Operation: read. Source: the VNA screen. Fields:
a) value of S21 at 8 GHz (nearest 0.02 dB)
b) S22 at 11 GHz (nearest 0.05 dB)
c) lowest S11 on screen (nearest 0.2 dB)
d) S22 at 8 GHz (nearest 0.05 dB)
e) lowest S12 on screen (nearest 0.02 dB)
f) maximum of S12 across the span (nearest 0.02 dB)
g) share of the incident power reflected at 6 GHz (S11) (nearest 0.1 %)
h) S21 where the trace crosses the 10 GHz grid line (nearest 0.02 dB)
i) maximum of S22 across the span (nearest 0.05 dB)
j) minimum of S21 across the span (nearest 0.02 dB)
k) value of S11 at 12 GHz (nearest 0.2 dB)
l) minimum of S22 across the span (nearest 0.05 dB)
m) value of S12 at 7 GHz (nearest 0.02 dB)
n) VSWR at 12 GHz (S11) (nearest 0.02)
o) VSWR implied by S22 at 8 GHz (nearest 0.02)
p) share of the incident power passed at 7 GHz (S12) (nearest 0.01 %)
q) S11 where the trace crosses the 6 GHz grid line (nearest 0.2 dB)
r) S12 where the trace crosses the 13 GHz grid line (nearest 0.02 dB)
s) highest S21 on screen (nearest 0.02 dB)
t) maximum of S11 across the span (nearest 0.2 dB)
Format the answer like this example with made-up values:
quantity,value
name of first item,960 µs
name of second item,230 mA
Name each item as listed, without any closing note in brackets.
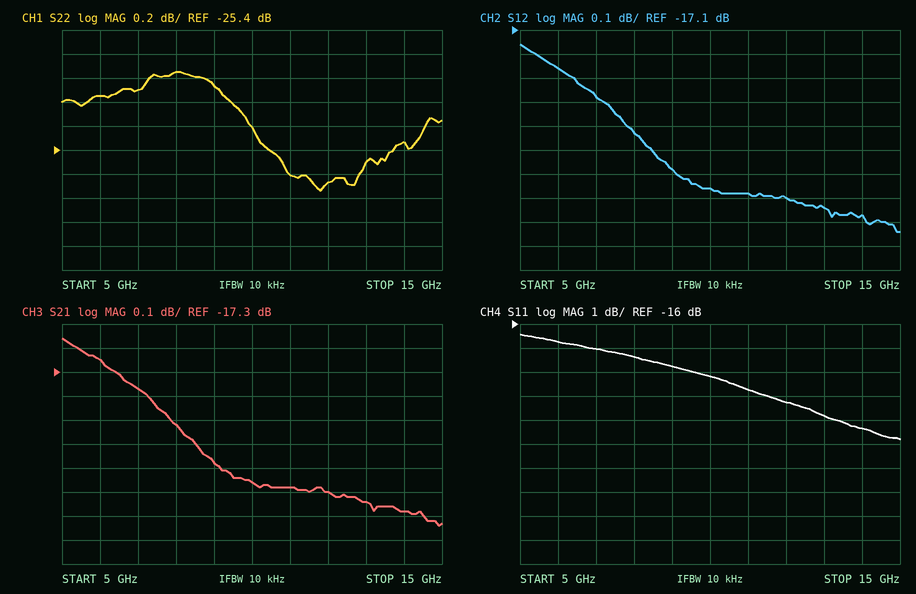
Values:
quantity,value
value of S21 at 8 GHz,-17.52 dB
S22 at 11 GHz,-25.60 dB
lowest S11 on screen,-20.8 dB
S22 at 8 GHz,-24.75 dB
lowest S12 on screen,-17.94 dB
maximum of S12 across the span,-17.16 dB
share of the incident power reflected at 6 GHz (S11),2.1 %
S21 where the trace crosses the 10 GHz grid line,-17.76 dB
maximum of S22 across the span,-24.75 dB
minimum of S21 across the span,-17.94 dB
value of S11 at 12 GHz,-19.2 dB
minimum of S22 across the span,-25.75 dB
value of S12 at 7 GHz,-17.38 dB
VSWR at 12 GHz (S11),1.24
VSWR implied by S22 at 8 GHz,1.12
share of the incident power passed at 7 GHz (S12),1.83 %
S11 where the trace crosses the 6 GHz grid line,-16.8 dB
S12 where the trace crosses the 13 GHz grid line,-17.84 dB
highest S21 on screen,-17.16 dB
maximum of S11 across the span,-16.4 dB
